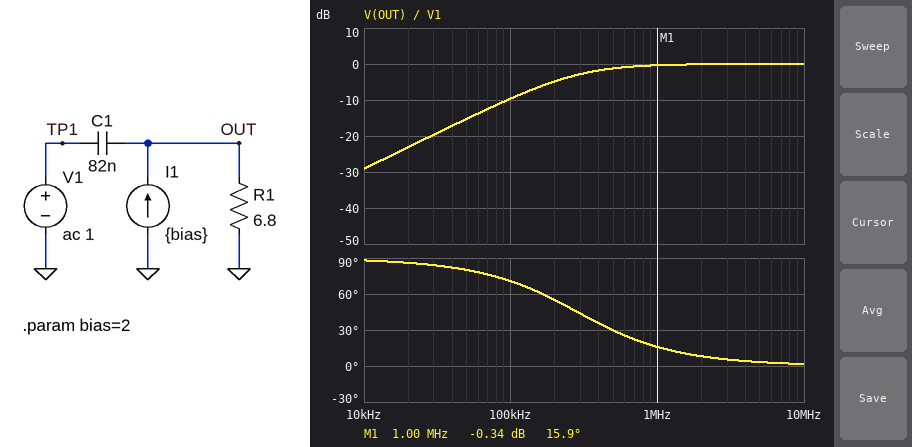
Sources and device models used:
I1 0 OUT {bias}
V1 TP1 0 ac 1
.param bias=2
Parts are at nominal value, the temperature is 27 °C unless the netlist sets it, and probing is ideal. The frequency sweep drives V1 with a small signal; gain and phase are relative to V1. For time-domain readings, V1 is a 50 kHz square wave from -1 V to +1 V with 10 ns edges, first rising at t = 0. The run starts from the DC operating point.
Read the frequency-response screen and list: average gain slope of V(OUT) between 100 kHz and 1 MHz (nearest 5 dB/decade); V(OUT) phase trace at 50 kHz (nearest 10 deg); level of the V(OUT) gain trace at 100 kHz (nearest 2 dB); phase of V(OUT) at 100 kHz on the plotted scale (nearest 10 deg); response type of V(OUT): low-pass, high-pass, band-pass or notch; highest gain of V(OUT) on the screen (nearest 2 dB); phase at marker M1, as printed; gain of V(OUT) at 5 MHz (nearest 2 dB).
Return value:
10 dB/decade
80 deg
-10 dB
70 deg
high-pass
0 dB
15.9 deg
0 dB
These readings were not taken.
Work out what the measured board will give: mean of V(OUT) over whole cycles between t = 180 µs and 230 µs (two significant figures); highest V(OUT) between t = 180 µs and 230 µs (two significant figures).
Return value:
14 V
16 V
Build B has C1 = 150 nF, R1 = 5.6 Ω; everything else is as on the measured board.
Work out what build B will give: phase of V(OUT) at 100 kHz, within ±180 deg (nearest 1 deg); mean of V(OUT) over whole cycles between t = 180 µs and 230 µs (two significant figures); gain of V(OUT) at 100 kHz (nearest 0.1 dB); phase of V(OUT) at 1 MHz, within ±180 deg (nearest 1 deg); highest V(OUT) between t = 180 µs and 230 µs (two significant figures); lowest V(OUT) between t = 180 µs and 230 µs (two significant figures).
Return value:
62 deg
11 V
-6.6 dB
11 deg
13 V
9.2 V
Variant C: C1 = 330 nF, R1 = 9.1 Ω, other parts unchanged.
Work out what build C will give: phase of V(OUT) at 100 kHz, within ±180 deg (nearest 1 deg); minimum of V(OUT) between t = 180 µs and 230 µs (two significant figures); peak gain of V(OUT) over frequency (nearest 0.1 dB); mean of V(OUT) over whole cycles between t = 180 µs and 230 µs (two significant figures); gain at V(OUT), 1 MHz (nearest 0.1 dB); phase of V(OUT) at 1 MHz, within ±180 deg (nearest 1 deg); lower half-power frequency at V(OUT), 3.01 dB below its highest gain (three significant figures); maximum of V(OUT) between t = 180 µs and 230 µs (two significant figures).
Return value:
28 deg
16 V
0 dB
18 V
0 dB
3 deg
53.0 kHz
20 V
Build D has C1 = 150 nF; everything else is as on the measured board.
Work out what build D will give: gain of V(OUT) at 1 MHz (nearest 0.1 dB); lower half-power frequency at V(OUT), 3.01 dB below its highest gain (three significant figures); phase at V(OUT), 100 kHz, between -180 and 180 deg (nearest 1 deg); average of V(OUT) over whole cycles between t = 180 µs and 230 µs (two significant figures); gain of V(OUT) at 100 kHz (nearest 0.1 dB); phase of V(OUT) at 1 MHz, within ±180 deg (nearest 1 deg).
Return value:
-0.1 dB
156 kHz
57 deg
14 V
-5.4 dB
9 deg
